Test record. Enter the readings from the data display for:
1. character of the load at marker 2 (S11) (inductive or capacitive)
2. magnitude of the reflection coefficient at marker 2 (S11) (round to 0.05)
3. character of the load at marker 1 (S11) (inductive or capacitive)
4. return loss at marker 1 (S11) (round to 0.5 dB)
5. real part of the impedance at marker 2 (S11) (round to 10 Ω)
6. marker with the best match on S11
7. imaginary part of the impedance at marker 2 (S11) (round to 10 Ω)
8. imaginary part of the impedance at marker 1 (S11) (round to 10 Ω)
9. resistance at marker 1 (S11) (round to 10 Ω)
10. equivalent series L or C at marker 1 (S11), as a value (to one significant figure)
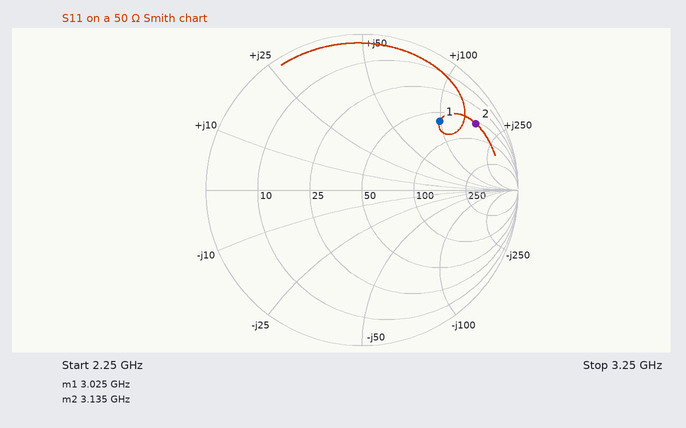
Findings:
inductive
0.85
inductive
3.5 dB
60 Ω
marker 1
+170 Ω
+100 Ω
60 Ω
5 nH
